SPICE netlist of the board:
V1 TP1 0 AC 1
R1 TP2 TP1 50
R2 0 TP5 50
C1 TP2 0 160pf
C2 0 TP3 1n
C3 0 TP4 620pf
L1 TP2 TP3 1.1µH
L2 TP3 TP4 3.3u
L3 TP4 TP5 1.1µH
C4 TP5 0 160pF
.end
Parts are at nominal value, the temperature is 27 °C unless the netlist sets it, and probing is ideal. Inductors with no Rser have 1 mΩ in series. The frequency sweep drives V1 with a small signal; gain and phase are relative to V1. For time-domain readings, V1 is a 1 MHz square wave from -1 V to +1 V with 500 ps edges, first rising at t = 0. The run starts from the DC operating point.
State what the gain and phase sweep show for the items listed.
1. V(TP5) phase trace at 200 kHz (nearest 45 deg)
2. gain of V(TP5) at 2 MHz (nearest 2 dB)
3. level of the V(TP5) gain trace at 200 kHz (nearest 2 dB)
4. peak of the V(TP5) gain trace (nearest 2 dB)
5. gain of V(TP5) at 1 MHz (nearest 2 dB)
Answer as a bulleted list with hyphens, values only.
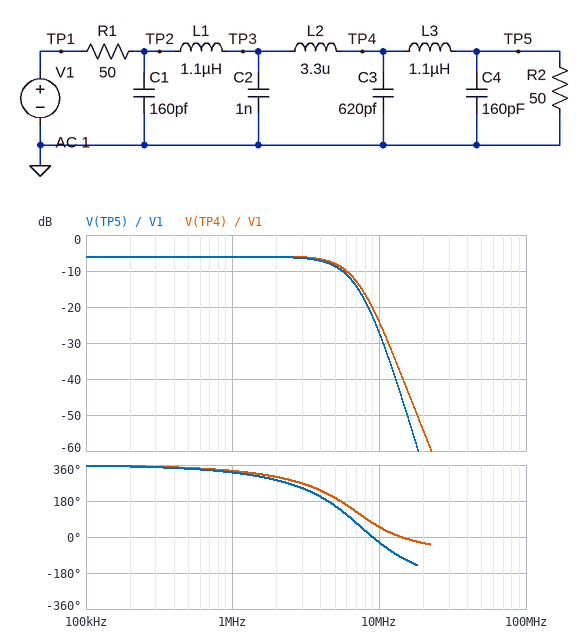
- 360 deg
- -6 dB
- -6 dB
- -6 dB
- -6 dB
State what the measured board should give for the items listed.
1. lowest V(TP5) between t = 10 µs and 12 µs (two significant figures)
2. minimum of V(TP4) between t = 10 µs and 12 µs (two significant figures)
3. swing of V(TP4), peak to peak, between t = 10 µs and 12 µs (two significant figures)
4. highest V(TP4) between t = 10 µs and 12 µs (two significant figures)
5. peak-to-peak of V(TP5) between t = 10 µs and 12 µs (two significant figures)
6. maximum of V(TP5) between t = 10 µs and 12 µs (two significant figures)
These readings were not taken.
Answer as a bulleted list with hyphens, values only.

- -580 mV
- -590 mV
- 1.2 V
- 590 mV
- 1.2 V
- 580 mV
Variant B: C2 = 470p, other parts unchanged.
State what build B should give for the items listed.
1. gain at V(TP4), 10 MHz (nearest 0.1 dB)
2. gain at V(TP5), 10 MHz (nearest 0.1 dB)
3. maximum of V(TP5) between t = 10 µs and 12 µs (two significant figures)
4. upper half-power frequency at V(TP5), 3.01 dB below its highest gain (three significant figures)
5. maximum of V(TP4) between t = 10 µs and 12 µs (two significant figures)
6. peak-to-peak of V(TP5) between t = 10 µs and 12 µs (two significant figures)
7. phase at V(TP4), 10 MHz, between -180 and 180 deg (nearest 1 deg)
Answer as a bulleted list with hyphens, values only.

- -14.8 dB
- -17.8 dB
- 560 mV
- 6.73 MHz
- 580 mV
- 1.1 V
- 79 deg
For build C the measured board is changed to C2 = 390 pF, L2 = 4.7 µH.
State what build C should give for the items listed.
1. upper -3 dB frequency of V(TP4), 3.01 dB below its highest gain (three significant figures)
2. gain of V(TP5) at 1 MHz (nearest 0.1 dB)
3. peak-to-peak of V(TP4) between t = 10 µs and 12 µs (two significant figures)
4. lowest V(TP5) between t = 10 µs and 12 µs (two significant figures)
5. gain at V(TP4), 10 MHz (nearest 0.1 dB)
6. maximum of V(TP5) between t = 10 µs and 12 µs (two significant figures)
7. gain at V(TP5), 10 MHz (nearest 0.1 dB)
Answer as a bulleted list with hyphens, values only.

- 4.98 MHz
- -6.2 dB
- 1.0 V
- -500 mV
- -16.9 dB
- 500 mV
- -19.9 dB
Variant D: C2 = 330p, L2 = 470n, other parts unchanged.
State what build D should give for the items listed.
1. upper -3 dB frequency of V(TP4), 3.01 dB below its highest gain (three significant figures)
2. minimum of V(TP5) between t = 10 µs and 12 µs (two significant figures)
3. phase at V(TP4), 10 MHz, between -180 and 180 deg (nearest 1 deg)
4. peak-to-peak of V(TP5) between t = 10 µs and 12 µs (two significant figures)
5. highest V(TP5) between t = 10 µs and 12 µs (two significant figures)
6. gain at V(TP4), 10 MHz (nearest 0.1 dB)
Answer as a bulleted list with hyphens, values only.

- 18.4 MHz
- -560 mV
- -151 deg
- 1.1 V
- 560 mV
- -7.3 dB
